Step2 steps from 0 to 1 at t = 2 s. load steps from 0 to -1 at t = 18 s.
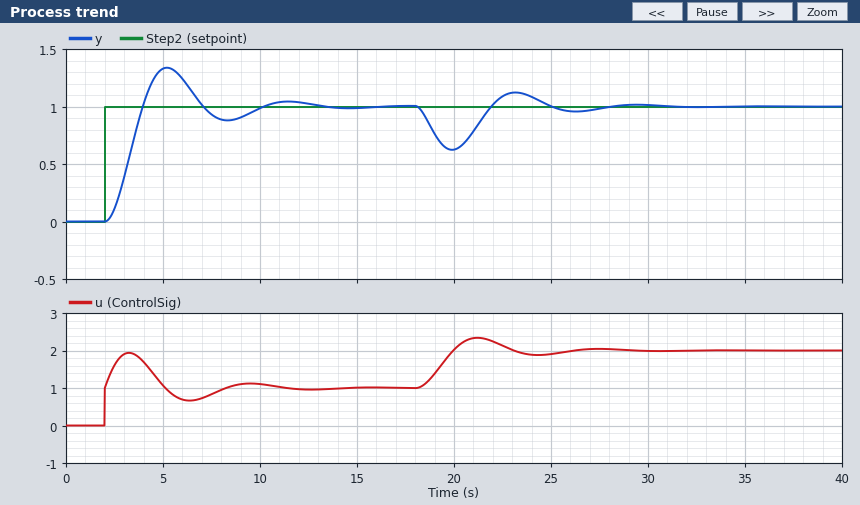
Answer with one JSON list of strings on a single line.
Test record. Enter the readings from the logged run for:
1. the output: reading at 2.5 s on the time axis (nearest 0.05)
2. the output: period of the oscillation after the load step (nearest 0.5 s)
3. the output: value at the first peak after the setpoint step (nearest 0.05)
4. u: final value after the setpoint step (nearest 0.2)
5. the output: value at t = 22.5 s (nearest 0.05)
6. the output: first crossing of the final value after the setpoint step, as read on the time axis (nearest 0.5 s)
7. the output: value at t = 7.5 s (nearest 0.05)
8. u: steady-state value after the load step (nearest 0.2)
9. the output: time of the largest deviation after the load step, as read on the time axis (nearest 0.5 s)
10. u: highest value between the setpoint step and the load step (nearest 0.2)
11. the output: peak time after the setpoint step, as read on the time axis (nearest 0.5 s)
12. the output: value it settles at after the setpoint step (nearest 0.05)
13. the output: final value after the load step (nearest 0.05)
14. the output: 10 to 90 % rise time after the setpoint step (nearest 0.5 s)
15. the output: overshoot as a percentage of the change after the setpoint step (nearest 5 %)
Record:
["0.10", "6.5 s", "1.35", "1.0", "1.10", "4.0 s", "0.95", "2.0", "20.0 s", "2.0", "5.0 s", "1.00", "1.00", "1.5 s", "35 %"]
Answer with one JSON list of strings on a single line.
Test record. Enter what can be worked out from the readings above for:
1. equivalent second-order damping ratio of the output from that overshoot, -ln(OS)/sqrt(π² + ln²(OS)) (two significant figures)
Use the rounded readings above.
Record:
["0.32"]
